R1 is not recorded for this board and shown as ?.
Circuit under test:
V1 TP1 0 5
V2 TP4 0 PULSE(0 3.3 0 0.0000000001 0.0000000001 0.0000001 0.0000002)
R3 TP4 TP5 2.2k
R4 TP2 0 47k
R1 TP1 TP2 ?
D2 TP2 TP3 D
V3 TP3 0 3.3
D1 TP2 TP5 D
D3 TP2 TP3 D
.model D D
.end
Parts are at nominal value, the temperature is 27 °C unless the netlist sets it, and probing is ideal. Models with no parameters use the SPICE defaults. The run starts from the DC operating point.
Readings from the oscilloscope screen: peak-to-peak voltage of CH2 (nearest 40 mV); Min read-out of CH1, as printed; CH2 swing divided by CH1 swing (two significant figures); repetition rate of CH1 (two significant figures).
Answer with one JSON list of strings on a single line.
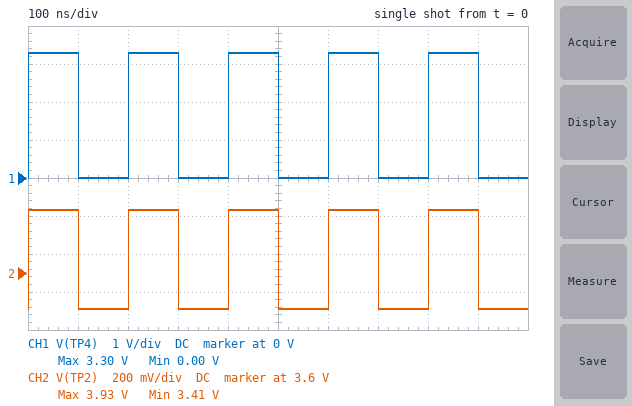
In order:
["520 mV", "0.00 V", "0.16", "5.0 MHz"]
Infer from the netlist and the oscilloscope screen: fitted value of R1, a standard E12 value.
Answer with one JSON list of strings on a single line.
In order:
["1.2 kΩ"]
